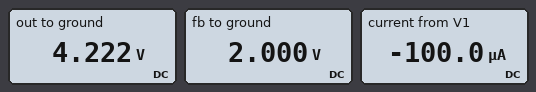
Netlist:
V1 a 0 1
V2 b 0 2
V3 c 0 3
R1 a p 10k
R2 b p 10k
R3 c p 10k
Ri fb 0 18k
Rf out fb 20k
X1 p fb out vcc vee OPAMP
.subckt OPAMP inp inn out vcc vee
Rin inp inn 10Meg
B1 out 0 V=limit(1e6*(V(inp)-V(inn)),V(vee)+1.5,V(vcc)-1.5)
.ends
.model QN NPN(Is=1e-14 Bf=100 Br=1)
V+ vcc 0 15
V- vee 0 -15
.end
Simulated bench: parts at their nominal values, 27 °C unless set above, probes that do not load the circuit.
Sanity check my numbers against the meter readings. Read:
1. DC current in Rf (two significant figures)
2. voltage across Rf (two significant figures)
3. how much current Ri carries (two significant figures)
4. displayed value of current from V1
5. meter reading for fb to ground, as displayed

110 µA
2.2 V
110 µA
-100.0 µA
2.000 V
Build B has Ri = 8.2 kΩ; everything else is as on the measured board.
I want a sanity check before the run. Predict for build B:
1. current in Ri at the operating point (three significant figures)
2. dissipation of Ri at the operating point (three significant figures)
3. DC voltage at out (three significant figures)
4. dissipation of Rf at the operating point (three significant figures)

244 µA
488 µW
6.88 V
1.19 mW
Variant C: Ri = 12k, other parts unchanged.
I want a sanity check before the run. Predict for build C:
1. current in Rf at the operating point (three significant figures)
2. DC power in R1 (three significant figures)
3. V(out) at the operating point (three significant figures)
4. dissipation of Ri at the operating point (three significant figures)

167 µA
100 µW
5.33 V
333 µW
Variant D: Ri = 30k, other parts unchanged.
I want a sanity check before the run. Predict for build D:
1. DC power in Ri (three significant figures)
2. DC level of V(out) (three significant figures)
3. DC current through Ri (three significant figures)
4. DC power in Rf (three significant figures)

133 µW
3.33 V
66.7 µA
88.9 µW
